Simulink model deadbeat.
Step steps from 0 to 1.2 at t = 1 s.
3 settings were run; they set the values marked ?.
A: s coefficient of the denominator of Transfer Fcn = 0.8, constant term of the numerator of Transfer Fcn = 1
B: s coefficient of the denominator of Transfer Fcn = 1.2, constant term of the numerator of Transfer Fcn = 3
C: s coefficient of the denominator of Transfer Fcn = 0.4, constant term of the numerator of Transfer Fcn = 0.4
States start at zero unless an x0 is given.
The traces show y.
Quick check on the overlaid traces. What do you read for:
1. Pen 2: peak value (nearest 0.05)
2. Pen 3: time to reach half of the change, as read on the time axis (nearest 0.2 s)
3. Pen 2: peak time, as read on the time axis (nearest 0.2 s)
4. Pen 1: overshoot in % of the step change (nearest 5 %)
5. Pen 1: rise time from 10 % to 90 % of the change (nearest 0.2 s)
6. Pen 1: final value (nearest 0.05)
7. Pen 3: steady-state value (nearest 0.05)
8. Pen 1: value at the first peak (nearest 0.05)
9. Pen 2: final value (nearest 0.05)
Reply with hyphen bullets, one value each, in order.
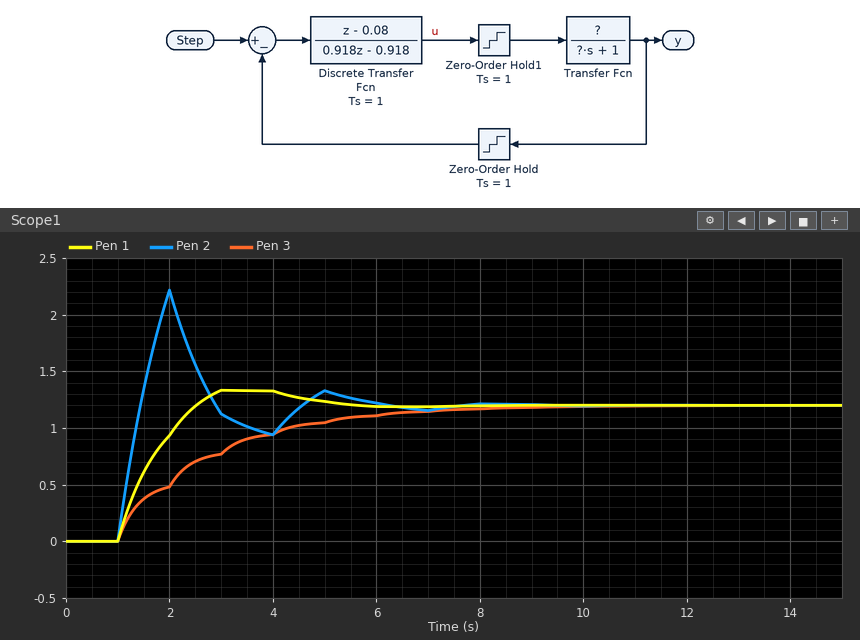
- 2.20
- 2.2 s
- 2.0 s
- 10 %
- 1.2 s
- 1.20
- 1.20
- 1.35
- 1.20
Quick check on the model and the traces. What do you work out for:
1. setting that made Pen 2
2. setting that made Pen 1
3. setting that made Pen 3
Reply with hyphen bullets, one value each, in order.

- B
- A
- C
